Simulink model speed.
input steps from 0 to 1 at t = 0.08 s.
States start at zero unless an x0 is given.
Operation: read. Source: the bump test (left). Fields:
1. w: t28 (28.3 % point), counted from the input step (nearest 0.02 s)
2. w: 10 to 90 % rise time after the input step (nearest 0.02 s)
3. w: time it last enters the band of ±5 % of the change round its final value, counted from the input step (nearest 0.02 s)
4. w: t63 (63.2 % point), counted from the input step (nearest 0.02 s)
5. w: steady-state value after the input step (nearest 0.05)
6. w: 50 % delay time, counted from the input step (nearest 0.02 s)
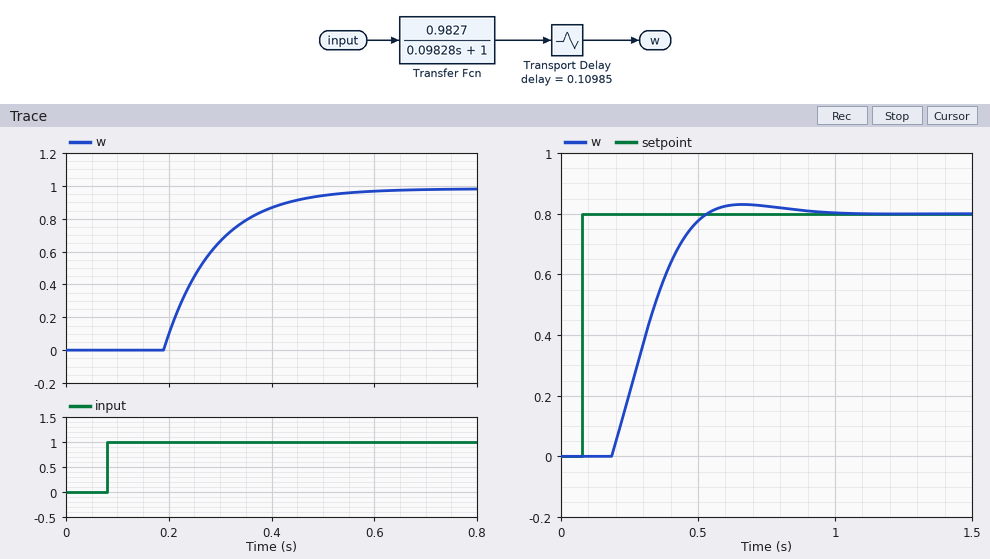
0.14 s
0.22 s
0.40 s
0.20 s
1.00
0.18 s
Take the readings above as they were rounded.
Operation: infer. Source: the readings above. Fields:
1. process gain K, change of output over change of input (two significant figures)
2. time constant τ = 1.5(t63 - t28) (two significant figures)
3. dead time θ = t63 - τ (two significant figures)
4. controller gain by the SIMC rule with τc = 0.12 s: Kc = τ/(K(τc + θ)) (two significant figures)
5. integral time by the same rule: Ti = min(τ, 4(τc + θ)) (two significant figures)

1.0
0.090 s
0.11 s
0.39
0.090 s
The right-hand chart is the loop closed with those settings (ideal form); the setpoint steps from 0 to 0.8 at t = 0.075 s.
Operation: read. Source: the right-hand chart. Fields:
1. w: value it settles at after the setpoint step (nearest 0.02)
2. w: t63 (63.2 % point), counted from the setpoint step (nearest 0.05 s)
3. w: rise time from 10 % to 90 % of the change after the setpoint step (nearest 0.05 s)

0.80
0.25 s
0.25 s
